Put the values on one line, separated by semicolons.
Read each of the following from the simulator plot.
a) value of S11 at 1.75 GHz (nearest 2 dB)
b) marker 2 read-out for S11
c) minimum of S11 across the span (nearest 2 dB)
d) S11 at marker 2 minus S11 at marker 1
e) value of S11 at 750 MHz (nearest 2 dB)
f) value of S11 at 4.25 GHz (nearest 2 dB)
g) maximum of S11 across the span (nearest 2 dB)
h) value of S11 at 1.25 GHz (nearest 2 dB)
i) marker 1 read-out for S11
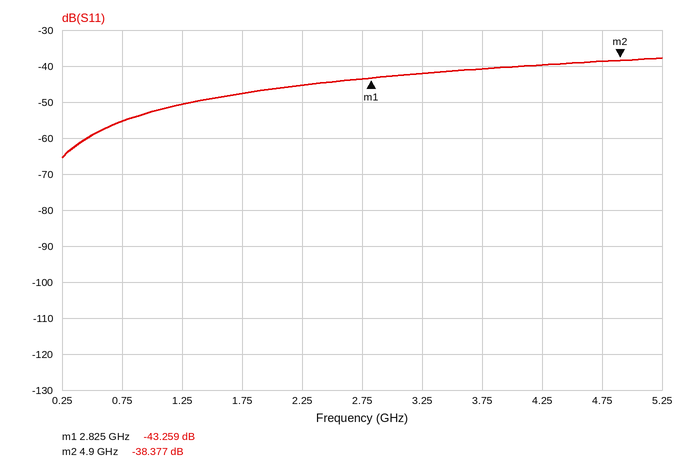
-48 dB; -38.377 dB; -66 dB; 4.882 dB; -56 dB; -40 dB; -38 dB; -50 dB; -43.259 dB
